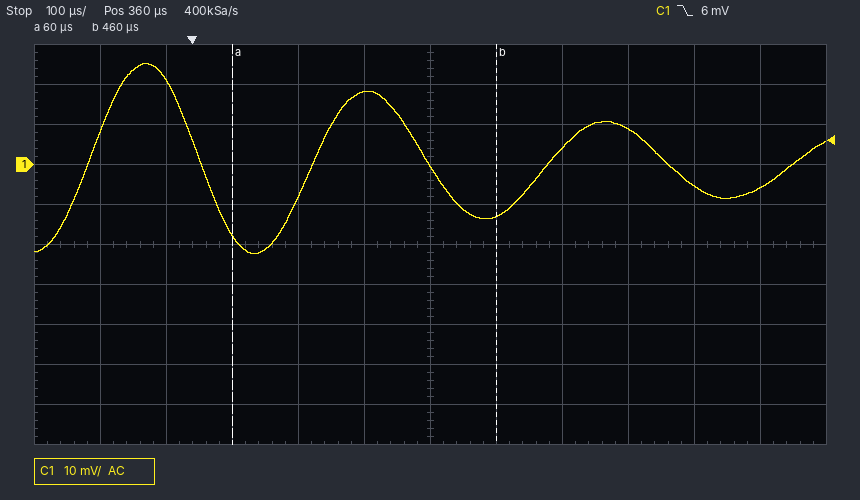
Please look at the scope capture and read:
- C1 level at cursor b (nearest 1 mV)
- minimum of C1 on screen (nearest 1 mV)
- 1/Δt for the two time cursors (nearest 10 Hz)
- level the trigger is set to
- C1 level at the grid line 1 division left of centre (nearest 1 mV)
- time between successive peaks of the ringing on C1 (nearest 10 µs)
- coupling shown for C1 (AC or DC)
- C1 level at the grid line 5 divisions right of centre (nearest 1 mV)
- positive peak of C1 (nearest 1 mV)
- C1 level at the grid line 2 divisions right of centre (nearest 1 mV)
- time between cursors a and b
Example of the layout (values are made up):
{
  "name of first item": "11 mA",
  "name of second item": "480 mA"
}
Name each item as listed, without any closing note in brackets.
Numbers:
{
  "C1 level at cursor b": "-13 mV",
  "minimum of C1 on screen": "-22 mV",
  "1/Δt for the two time cursors": "2.50 kHz",
  "level the trigger is set to": "6 mV",
  "C1 level at the grid line 1 division left of centre": "18 mV",
  "time between successive peaks of the ringing on C1": "350 µs",
  "coupling shown for C1": "AC",
  "C1 level at the grid line 5 divisions right of centre": "-6 mV",
  "positive peak of C1": "25 mV",
  "C1 level at the grid line 2 divisions right of centre": "4 mV",
  "time between cursors a and b": "400 µs"
}
